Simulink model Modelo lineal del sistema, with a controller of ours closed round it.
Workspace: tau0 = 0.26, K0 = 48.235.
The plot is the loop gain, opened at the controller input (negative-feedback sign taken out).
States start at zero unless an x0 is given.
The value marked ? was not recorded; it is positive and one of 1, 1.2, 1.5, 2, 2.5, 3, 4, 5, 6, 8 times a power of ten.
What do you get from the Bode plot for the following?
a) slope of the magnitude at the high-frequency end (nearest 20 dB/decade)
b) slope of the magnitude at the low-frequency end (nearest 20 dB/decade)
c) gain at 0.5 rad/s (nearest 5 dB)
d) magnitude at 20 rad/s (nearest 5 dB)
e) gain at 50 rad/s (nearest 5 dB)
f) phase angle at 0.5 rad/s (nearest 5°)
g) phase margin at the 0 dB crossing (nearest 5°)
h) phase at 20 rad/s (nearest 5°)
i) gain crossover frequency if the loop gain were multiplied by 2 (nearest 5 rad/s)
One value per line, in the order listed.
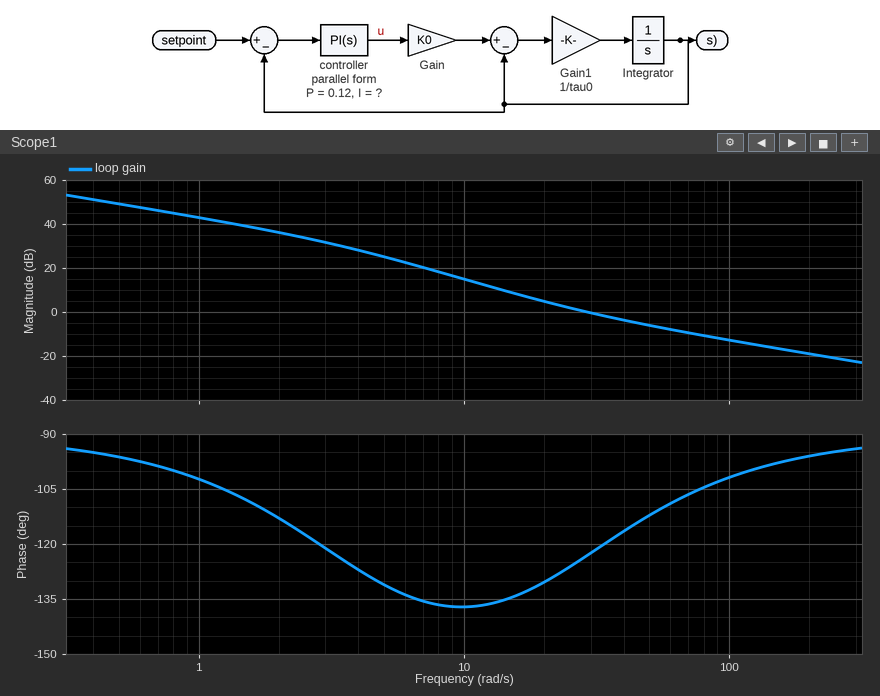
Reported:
-20 dB/decade
-20 dB/decade
50 dB
5 dB
-5 dB
-95°
55°
-130°
50 rad/s
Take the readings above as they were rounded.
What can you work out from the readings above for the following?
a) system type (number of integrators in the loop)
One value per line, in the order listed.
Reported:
1
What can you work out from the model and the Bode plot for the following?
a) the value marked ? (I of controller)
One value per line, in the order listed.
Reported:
3
